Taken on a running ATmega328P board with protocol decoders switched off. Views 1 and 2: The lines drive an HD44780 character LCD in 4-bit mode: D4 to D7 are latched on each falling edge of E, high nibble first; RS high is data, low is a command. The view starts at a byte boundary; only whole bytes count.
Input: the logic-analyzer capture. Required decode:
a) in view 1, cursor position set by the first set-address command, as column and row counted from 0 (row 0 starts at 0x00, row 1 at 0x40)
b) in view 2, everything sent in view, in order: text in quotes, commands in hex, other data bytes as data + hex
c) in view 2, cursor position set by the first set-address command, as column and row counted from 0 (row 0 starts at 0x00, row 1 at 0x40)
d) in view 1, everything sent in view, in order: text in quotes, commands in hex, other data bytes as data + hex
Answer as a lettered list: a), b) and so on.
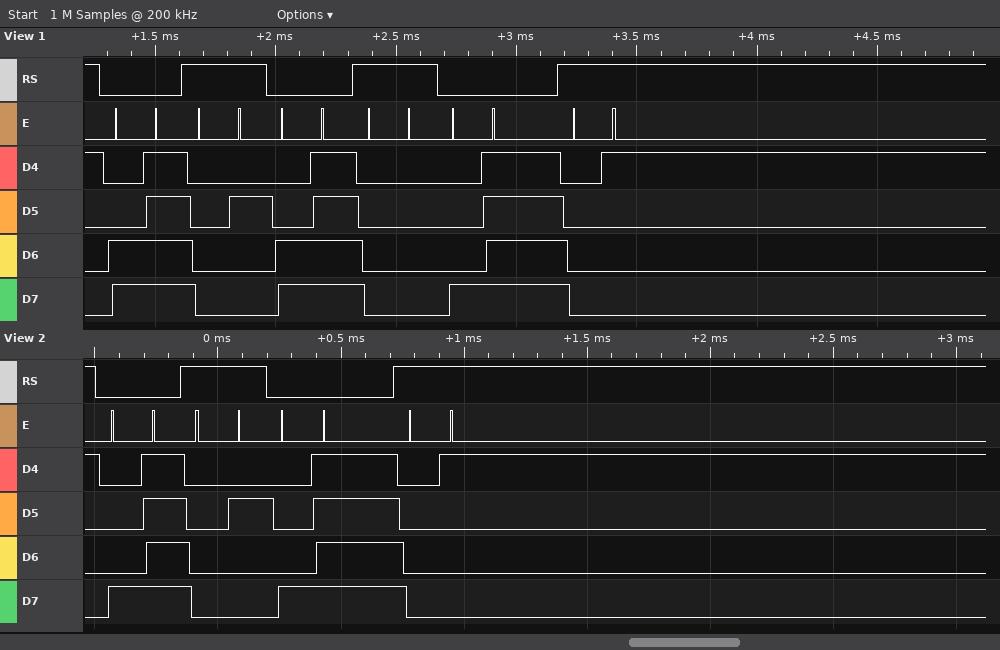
a) column 15, row 1
b) 0x8F data 02 0x8F data 01
c) column 15, row 0
d) 0xCF data 02 0xCF data 00 0x8F data 01
